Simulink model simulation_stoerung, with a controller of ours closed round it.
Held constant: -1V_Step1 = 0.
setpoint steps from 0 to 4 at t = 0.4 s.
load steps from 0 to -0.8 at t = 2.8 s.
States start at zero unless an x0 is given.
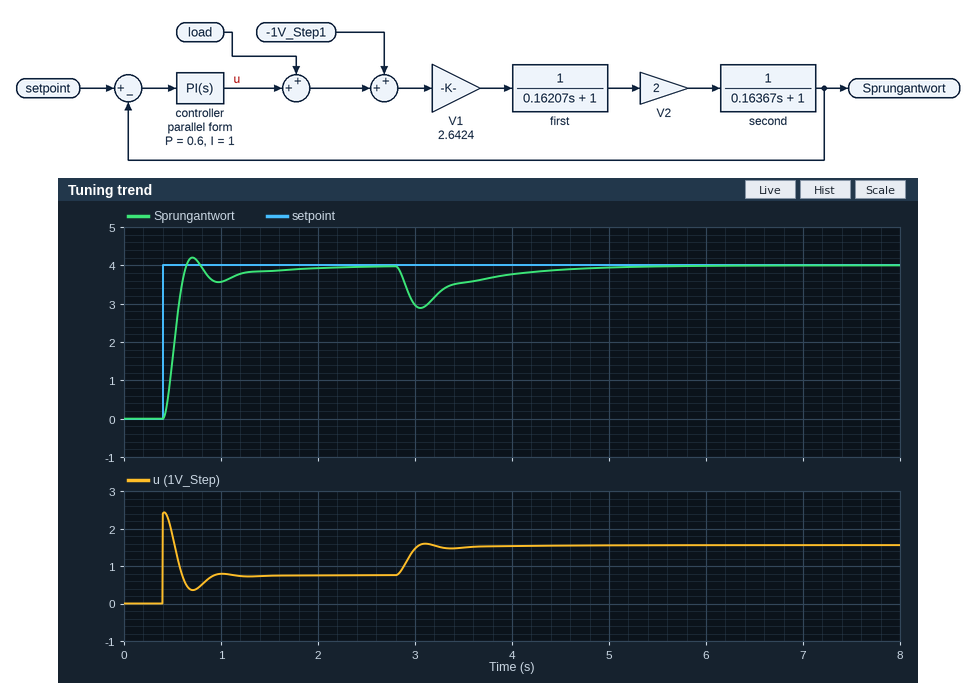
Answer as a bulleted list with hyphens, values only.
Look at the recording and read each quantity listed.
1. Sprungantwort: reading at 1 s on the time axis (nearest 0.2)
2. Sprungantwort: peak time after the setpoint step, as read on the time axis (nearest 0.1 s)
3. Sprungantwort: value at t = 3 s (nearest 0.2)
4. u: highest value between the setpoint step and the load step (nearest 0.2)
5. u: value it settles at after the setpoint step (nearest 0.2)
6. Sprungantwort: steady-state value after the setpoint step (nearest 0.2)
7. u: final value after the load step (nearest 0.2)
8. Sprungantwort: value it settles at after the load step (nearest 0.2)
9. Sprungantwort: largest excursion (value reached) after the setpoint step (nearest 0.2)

- 3.6
- 0.7 s
- 3.0
- 2.4
- 0.8
- 4.0
- 1.6
- 4.0
- 4.2
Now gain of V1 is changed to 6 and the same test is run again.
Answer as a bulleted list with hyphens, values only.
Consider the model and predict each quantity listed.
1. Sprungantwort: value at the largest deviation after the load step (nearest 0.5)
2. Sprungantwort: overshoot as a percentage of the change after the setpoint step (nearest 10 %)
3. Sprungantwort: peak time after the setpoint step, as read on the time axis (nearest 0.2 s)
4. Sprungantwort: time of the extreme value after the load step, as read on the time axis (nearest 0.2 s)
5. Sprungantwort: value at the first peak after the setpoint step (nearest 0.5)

- 2.5
- 30 %
- 0.6 s
- 3.0 s
- 5.0
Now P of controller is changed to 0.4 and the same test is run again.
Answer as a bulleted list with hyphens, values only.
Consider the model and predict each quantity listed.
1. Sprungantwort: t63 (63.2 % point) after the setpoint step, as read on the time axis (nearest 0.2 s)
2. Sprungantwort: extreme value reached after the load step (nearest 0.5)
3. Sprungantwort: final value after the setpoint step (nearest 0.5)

- 0.6 s
- 2.5
- 4.0
